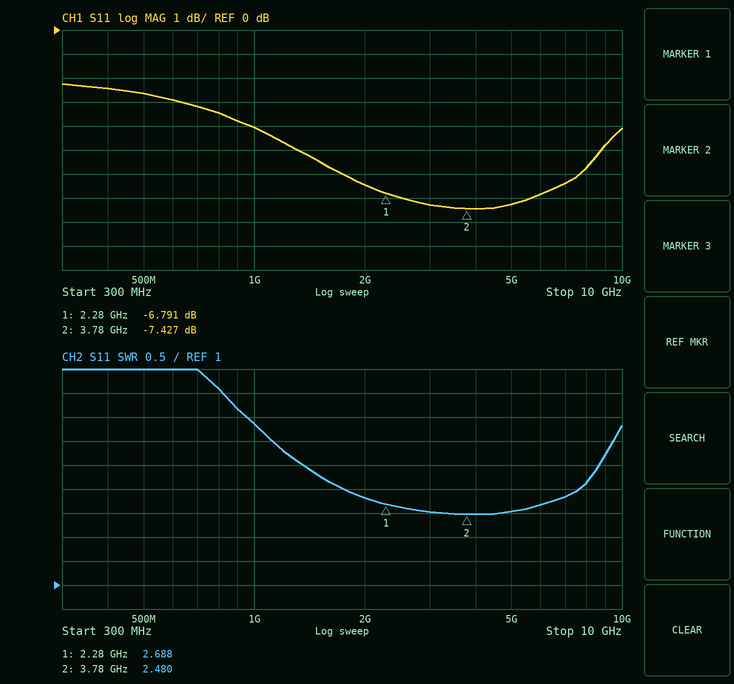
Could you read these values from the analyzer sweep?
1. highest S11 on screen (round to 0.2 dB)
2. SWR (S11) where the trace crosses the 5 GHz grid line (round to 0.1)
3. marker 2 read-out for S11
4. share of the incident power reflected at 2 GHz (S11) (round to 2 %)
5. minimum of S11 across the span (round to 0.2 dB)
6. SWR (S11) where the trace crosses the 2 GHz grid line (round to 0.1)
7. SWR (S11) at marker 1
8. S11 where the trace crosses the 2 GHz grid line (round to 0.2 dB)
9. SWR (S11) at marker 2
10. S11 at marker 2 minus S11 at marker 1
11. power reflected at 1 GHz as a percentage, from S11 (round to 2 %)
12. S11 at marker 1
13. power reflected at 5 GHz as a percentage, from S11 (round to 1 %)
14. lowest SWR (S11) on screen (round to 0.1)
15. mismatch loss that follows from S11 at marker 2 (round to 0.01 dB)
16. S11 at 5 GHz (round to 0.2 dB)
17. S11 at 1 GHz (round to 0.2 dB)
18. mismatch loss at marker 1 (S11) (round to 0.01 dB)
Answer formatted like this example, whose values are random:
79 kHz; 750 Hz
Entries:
-2.2 dB; 2.5; -7.427 dB; 22 %; -7.4 dB; 2.8; 2.688; -6.4 dB; 2.480; -0.636 dB; 40 %; -6.791 dB; 19 %; 2.5; 0.87 dB; -7.2 dB; -4.0 dB; 1.02 dB
